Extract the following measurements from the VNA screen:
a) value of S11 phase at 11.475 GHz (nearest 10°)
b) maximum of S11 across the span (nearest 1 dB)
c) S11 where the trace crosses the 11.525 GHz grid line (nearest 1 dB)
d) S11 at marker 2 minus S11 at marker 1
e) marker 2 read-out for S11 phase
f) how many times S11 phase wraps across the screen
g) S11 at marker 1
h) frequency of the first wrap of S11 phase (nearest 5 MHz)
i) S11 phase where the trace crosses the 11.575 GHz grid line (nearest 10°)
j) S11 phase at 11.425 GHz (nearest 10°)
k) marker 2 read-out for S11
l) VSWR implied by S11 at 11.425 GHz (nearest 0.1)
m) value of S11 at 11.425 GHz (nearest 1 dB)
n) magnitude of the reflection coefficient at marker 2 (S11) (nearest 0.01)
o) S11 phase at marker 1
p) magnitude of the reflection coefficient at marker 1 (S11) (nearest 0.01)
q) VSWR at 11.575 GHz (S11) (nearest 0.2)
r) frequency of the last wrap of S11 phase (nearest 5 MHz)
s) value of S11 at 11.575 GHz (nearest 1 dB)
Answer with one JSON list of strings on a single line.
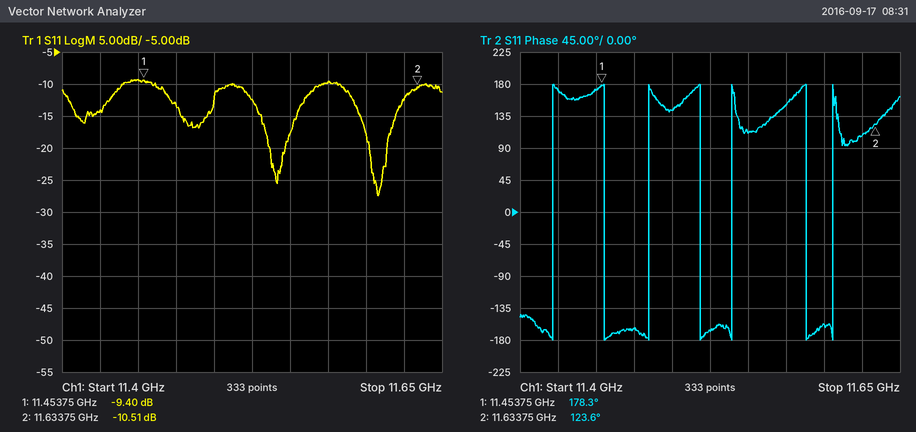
["-160°", "-9 dB", "-12 dB", "-1.11 dB", "123.6°", "7", "-9.40 dB", "11.420 GHz", "150°", "170°", "-10.51 dB", "1.5", "-14 dB", "0.30", "178.3°", "0.34", "2.0", "11.605 GHz", "-10 dB"]
